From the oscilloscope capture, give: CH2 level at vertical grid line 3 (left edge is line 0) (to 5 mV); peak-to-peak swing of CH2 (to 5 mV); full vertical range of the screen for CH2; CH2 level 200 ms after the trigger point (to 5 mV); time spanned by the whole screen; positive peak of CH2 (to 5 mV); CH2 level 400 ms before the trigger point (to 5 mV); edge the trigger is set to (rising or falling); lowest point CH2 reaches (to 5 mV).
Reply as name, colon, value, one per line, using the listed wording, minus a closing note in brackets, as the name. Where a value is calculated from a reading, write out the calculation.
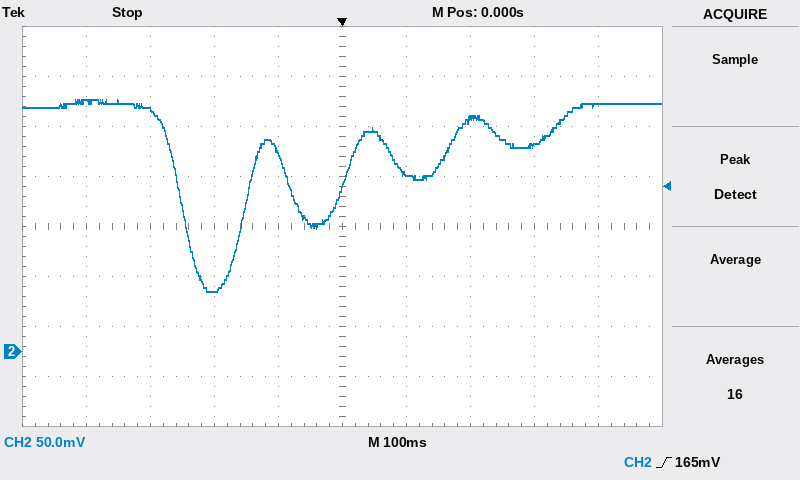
CH2 level at vertical grid line 3 (left edge is line 0): 60 mV
peak-to-peak swing of CH2: 250 mV − (60 mV) = 190 mV
full vertical range of the screen for CH2: 400 mV
CH2 level 200 ms after the trigger point: 230 mV
time spanned by the whole screen: 1 s
positive peak of CH2: 250 mV
CH2 level 400 ms before the trigger point: 250 mV
edge the trigger is set to: rising
lowest point CH2 reaches: 60 mV
